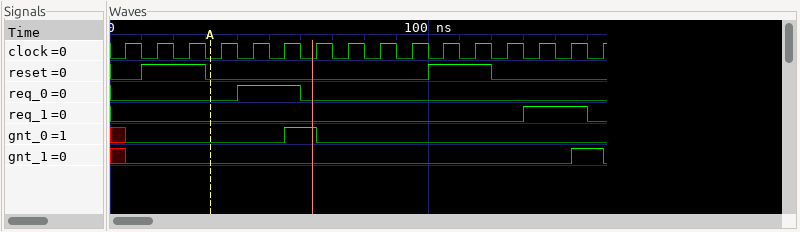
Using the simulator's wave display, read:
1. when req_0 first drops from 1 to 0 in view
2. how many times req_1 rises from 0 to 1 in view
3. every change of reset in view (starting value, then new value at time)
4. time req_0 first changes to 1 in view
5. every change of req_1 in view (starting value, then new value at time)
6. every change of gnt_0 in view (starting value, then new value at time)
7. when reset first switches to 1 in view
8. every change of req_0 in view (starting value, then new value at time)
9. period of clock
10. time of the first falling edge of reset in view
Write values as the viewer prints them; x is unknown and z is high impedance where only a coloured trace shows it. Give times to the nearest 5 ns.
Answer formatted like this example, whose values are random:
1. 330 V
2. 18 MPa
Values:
1. 60 ns
2. 1
3. 0, 1 at 10 ns, 0 at 30 ns, 1 at 100 ns, 0 at 120 ns
4. 40 ns
5. 0, 1 at 130 ns, 0 at 150 ns
6. x, 0 at 5 ns, 1 at 55 ns, 0 at 65 ns
7. 10 ns
8. 0, 1 at 40 ns, 0 at 60 ns
9. 10 ns
10. 30 ns
